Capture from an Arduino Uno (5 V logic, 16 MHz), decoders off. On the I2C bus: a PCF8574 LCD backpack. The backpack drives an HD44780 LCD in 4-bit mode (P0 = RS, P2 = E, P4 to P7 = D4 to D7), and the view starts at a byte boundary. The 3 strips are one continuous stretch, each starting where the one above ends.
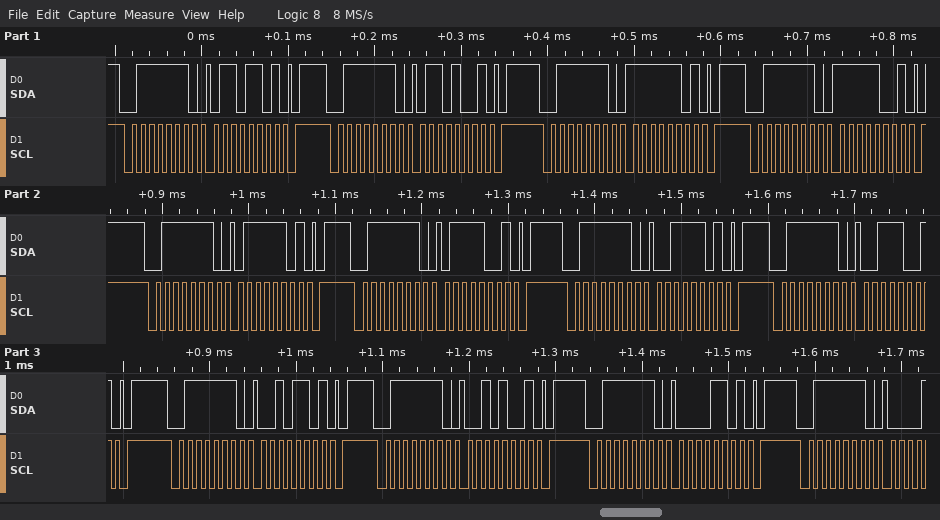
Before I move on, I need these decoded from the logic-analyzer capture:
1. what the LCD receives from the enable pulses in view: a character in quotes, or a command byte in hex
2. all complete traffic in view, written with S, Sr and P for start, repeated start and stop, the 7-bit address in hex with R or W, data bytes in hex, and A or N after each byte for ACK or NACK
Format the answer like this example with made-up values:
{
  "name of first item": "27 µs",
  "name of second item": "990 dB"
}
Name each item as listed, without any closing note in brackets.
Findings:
{
  "what the LCD receives from the enable pulses in view: a character in quotes, or a command byte in hex": "'o' 's'",
  "all complete traffic in view, written with S, Sr and P for start, repeated start and stop, the 7-bit address in hex with R or W, data bytes in hex, and A or N after each byte for ACK or NACK": "S 3FW A 6D A P S 3FW A 69 A P S 3FW A FD A P S 3FW A F9 A P S 3FW A 7D A P S 3FW A 79 A P S 3FW A 3D A P S 3FW A 39 A P S 3FW A 2D A P S 3FW A 29 A P S 3FW A 0D A P S 3FW A"
}
